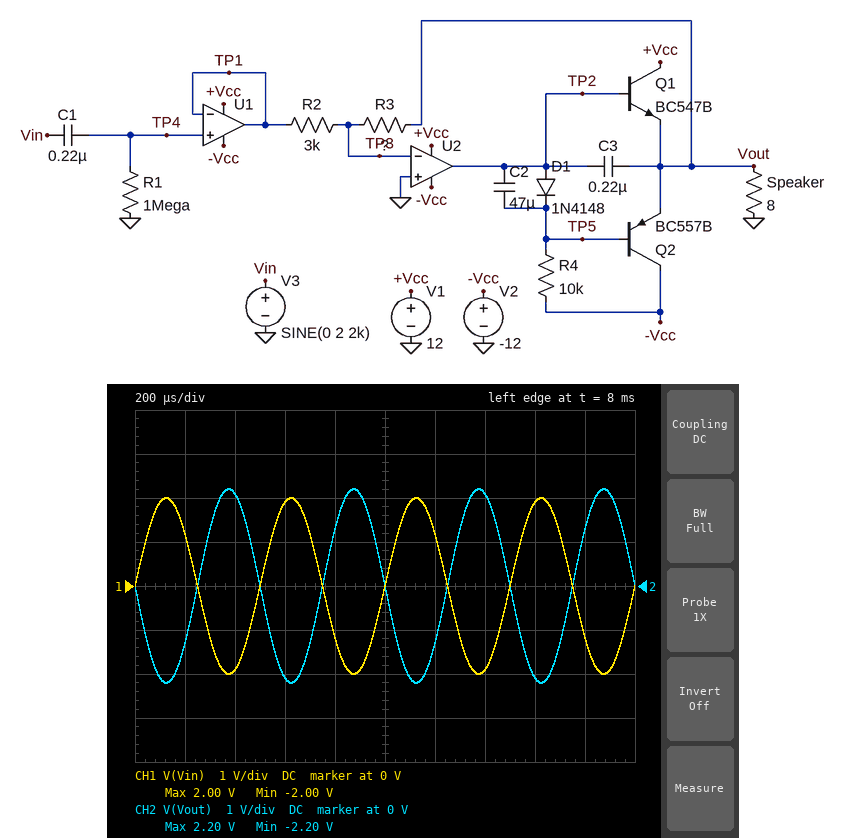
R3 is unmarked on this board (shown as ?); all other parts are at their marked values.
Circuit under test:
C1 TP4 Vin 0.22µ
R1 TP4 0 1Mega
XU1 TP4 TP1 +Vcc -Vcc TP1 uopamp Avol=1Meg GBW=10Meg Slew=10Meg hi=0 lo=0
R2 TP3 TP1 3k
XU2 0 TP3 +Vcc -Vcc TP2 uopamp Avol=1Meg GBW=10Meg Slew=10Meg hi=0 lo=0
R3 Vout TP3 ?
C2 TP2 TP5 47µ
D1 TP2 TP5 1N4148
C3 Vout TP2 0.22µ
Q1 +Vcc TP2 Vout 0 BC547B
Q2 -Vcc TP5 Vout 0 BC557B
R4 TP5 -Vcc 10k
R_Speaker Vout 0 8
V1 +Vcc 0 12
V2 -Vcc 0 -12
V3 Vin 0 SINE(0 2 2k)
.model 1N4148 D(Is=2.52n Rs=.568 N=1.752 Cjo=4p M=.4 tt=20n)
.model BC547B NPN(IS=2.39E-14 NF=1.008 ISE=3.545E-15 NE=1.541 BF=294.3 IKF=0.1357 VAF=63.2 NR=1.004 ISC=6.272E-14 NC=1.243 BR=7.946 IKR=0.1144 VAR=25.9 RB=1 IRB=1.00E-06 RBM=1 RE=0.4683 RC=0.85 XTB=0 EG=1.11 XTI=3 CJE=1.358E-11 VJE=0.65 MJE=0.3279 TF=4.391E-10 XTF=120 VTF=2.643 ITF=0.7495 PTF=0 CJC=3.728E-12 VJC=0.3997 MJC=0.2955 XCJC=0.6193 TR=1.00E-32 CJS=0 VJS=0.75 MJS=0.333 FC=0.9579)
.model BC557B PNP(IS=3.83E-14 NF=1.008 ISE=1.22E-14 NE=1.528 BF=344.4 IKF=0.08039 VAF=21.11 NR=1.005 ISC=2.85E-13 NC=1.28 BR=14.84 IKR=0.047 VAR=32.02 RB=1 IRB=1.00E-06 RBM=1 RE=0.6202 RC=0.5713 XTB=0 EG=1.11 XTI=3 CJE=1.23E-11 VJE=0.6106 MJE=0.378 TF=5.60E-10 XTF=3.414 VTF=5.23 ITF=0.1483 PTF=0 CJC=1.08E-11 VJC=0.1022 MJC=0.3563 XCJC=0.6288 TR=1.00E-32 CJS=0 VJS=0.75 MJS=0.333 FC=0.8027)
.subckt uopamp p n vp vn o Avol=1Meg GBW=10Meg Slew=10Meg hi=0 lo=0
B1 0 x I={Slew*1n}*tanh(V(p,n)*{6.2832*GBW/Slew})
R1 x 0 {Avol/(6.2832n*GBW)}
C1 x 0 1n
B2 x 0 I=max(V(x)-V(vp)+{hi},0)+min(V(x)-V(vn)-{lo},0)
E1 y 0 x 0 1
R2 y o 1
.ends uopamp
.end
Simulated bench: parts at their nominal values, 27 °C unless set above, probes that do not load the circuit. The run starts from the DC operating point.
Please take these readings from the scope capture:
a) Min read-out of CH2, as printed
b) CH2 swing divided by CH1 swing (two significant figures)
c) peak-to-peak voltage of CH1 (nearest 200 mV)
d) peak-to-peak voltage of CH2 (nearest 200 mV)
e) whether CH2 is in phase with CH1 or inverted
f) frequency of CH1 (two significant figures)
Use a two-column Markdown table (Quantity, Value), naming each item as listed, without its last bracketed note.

| Quantity | Value |
|---|---|
| Min read-out of CH2, as printed | -2.20 V |
| CH2 swing divided by CH1 swing | 1.1 |
| peak-to-peak voltage of CH1 | 4.0 V |
| peak-to-peak voltage of CH2 | 4.4 V |
| whether CH2 is in phase with CH1 or inverted | inverted |
| frequency of CH1 | 2.0 kHz |
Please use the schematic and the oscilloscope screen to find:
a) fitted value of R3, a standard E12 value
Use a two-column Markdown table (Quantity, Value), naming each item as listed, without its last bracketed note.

| Quantity | Value |
|---|---|
| fitted value of R3, a standard E12 value | 3.3 kΩ |
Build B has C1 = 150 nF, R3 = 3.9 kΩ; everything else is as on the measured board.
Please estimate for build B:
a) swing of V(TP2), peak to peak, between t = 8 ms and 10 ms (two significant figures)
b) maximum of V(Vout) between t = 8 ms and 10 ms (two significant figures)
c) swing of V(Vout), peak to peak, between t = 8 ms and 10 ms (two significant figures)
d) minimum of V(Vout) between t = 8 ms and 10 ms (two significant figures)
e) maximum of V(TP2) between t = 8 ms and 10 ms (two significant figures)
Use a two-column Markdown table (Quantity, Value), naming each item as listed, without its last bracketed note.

| Quantity | Value |
|---|---|
| swing of V(TP2), peak to peak, between t = 8 ms and 10 ms | 6.6 V |
| maximum of V(Vout) between t = 8 ms and 10 ms | 2.6 V |
| swing of V(Vout), peak to peak, between t = 8 ms and 10 ms | 5.2 V |
| minimum of V(Vout) between t = 8 ms and 10 ms | -2.6 V |
| maximum of V(TP2) between t = 8 ms and 10 ms | 3.6 V |
